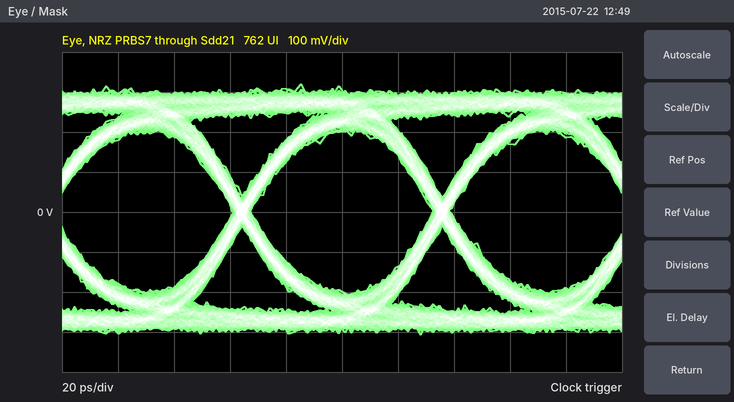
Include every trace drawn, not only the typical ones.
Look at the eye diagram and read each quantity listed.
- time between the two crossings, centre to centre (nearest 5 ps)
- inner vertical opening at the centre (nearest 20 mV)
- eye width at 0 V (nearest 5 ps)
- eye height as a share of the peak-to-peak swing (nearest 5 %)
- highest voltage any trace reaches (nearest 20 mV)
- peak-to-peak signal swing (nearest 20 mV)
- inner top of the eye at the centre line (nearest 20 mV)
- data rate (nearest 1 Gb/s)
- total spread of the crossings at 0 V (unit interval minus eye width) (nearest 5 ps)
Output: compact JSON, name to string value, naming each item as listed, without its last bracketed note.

{"time between the two crossings, centre to centre": "70 ps", "inner vertical opening at the centre": "400 mV", "eye width at 0 V": "65 ps", "eye height as a share of the peak-to-peak swing": "65 %", "highest voltage any trace reaches": "320 mV", "peak-to-peak signal swing": "620 mV", "inner top of the eye at the centre line": "200 mV", "data rate": "14 Gb/s", "total spread of the crossings at 0 V (unit interval minus eye width)": "5 ps"}
